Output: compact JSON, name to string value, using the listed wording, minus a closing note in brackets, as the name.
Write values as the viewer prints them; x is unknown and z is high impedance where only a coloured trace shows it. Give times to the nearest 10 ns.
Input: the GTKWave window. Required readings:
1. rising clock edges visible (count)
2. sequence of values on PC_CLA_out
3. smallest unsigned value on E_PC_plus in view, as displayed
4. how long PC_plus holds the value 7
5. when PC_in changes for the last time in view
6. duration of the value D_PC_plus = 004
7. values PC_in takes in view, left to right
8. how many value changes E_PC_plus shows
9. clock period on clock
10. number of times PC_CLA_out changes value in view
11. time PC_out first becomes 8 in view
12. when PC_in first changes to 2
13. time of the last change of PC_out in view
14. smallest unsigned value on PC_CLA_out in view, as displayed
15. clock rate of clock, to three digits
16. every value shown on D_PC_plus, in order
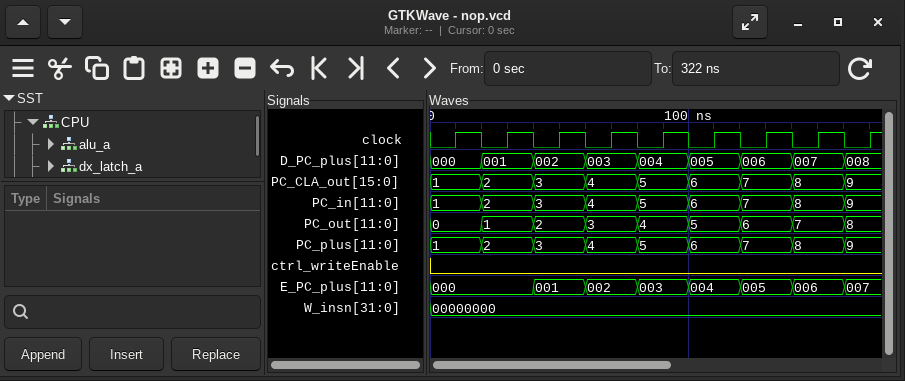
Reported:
{"rising clock edges visible": "9", "sequence of values on PC_CLA_out": "1, 2, 3, 4, 5, 6, 7, 8, 9", "smallest unsigned value on E_PC_plus in view, as displayed": "000", "how long PC_plus holds the value 7": "20 ns", "when PC_in changes for the last time in view": "160 ns", "duration of the value D_PC_plus = 004": "20 ns", "values PC_in takes in view, left to right": "1, 2, 3, 4, 5, 6, 7, 8, 9", "how many value changes E_PC_plus shows": "7", "clock period on clock": "20 ns", "number of times PC_CLA_out changes value in view": "8", "time PC_out first becomes 8 in view": "160 ns", "when PC_in first changes to 2": "20 ns", "time of the last change of PC_out in view": "160 ns", "smallest unsigned value on PC_CLA_out in view, as displayed": "1", "clock rate of clock, to three digits": "50.0 MHz", "every value shown on D_PC_plus, in order": "000, 001, 002, 003, 004, 005, 006, 007, 008"}
